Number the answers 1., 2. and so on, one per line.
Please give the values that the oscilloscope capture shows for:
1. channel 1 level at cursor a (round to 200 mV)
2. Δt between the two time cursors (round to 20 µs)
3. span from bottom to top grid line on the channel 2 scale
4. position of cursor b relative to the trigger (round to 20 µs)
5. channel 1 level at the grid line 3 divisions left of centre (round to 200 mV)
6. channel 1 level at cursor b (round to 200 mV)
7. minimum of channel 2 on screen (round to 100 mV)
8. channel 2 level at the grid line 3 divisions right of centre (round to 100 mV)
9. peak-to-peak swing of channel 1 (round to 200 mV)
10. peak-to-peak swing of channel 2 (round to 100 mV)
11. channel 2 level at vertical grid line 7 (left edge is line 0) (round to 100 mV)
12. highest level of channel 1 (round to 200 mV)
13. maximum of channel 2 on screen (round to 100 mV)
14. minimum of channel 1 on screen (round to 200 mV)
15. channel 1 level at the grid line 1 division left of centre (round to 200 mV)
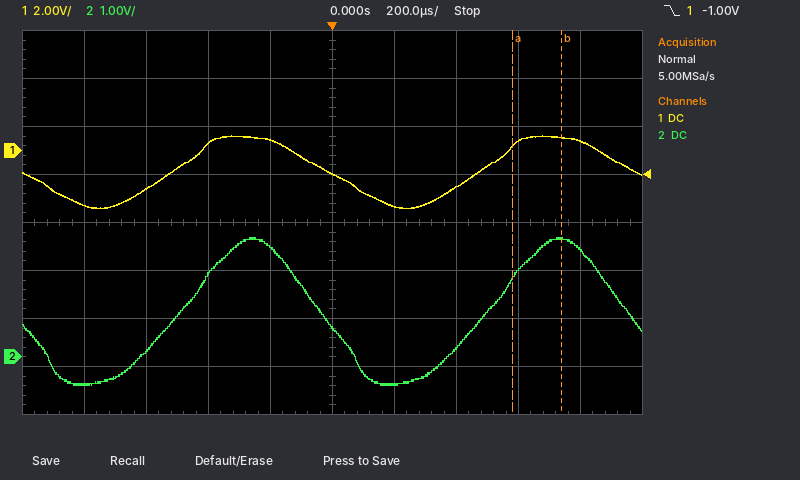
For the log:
1. 200 mV
2. 160 µs
3. 8 V
4. +740 µs
5. -1.6 V
6. 600 mV
7. -600 mV
8. 1.8 V
9. 3.0 V
10. 3.1 V
11. 200 mV
12. 600 mV
13. 2.5 V
14. -2.4 V
15. 400 mV
